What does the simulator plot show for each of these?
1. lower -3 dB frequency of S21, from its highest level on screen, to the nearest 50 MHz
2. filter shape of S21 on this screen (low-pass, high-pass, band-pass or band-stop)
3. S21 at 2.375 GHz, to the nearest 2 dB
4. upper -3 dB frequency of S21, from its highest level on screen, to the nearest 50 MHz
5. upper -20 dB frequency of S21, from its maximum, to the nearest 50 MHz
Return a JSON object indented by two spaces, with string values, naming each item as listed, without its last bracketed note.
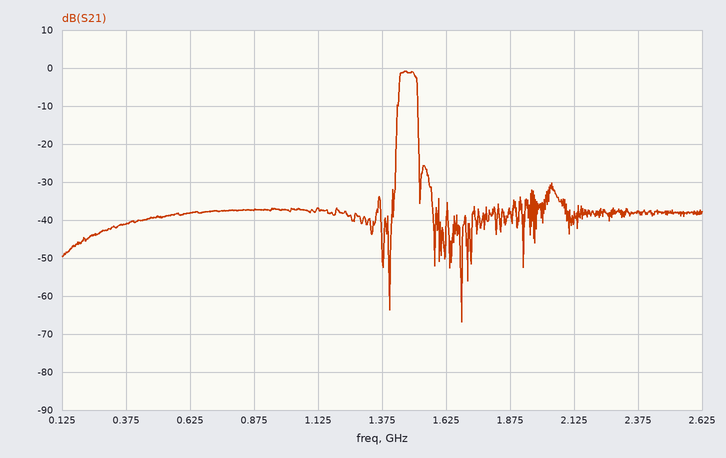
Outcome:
{
  "lower -3 dB frequency of S21, from its highest level on screen, to the nearest 50 MHz": "1.45 GHz",
  "filter shape of S21 on this screen": "band-pass",
  "S21 at 2.375 GHz, to the nearest 2 dB": "-38 dB",
  "upper -3 dB frequency of S21, from its highest level on screen, to the nearest 50 MHz": "1.50 GHz",
  "upper -20 dB frequency of S21, from its maximum, to the nearest 50 MHz": "1.50 GHz"
}
